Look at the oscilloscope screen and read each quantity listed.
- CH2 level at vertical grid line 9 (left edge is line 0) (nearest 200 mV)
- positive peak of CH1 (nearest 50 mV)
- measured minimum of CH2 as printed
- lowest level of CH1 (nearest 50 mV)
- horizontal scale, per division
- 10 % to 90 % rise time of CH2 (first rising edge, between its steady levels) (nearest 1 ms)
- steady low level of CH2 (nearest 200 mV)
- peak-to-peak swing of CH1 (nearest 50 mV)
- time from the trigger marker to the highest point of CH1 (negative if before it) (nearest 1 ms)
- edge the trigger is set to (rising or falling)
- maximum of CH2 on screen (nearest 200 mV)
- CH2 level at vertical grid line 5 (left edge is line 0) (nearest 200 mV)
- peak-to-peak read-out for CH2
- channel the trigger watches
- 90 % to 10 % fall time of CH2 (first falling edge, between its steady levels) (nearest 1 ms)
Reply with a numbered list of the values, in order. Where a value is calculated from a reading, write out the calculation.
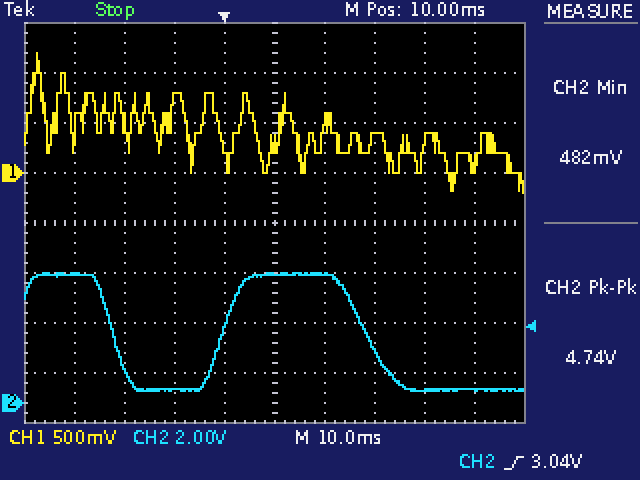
1. 600 mV
2. 1.20 V
3. 482 mV
4. -200 mV
5. 10 ms
6. 7 ms
7. 600 mV
8. 1.20 V − (-200 mV) = 1.40 V
9. -37 ms
10. rising
11. 5.2 V
12. 5.2 V
13. 4.74 V
14. CH2
15. 6 ms
